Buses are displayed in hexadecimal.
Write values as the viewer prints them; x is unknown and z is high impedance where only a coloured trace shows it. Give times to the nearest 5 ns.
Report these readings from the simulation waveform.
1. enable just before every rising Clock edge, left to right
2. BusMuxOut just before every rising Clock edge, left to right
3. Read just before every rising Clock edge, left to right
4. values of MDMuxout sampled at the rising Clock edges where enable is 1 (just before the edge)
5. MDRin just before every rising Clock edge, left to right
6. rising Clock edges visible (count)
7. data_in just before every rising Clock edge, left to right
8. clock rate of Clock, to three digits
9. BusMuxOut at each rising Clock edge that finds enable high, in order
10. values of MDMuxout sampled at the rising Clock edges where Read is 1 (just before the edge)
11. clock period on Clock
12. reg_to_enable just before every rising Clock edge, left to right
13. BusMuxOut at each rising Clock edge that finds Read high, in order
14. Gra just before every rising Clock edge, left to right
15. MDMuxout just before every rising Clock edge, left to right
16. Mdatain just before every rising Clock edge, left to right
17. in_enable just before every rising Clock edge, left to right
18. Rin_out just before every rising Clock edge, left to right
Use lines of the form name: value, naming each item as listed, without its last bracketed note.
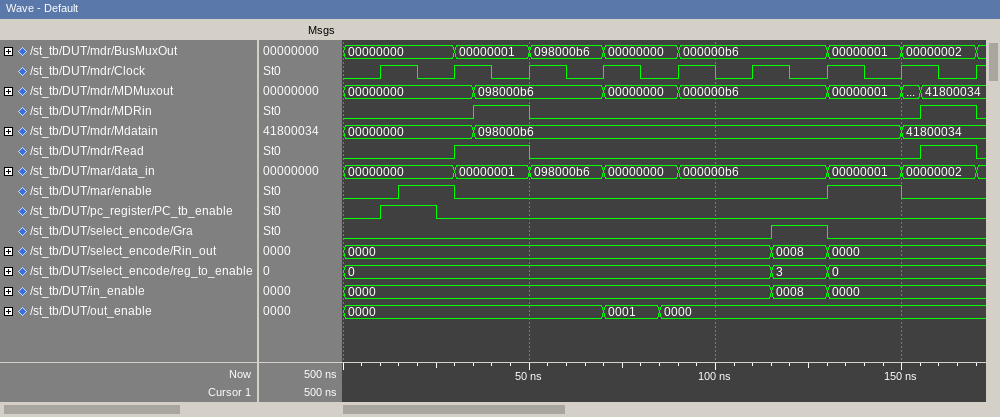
enable just before every rising Clock edge, left to right: 0 1 0 0 0 0 0 1 0
BusMuxOut just before every rising Clock edge, left to right: 00000000, 00000000, 00000001, 098000b6, 00000000, 000000b6, 000000b6, 00000001, 00000002
Read just before every rising Clock edge, left to right: 0 0 1 0 0 0 0 0 1
values of MDMuxout sampled at the rising Clock edges where enable is 1: 00000000, 00000001
MDRin just before every rising Clock edge, left to right: 0 0 1 0 0 0 0 0 1
rising Clock edges visible: 9
data_in just before every rising Clock edge, left to right: 00000000, 00000000, 00000001, 098000b6, 00000000, 000000b6, 000000b6, 00000001, 00000002
clock rate of Clock, to three digits: 50.0 MHz
BusMuxOut at each rising Clock edge that finds enable high, in order: 00000000, 00000001
values of MDMuxout sampled at the rising Clock edges where Read is 1: 098000b6, 41800034
clock period on Clock: 20 ns
reg_to_enable just before every rising Clock edge, left to right: 0, 0, 0, 0, 0, 0, 3, 0, 0
BusMuxOut at each rising Clock edge that finds Read high, in order: 00000001, 00000002
Gra just before every rising Clock edge, left to right: 0 0 0 0 0 0 1 0 0
MDMuxout just before every rising Clock edge, left to right: 00000000, 00000000, 098000b6, 098000b6, 00000000, 000000b6, 000000b6, 00000001, 41800034
Mdatain just before every rising Clock edge, left to right: 00000000, 00000000, 098000b6, 098000b6, 098000b6, 098000b6, 098000b6, 098000b6, 41800034
in_enable just before every rising Clock edge, left to right: 0000, 0000, 0000, 0000, 0000, 0000, 0008, 0000, 0000
Rin_out just before every rising Clock edge, left to right: 0000, 0000, 0000, 0000, 0000, 0000, 0008, 0000, 0000
